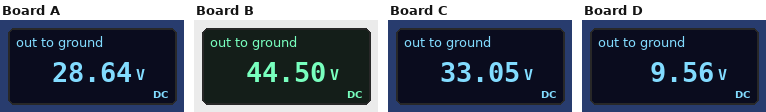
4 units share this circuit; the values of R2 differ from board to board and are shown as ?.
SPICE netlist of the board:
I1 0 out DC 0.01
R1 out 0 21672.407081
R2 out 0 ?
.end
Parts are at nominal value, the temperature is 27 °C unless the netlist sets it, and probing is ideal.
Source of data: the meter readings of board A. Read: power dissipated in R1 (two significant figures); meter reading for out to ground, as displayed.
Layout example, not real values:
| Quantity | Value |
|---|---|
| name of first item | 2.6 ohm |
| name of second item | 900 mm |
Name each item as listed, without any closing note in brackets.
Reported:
| Quantity | Value |
|---|---|
| power dissipated in R1 | 38 mW |
| meter reading for out to ground, as displayed | 28.64 V |
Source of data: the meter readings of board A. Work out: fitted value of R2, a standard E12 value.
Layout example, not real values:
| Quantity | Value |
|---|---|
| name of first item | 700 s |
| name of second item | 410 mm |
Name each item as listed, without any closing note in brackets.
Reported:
| Quantity | Value |
|---|---|
| fitted value of R2, a standard E12 value | 3.3 kΩ |
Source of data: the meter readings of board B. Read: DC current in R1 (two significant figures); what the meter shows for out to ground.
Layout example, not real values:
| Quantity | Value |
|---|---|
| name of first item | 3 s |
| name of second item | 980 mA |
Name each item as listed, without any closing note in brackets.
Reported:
| Quantity | Value |
|---|---|
| DC current in R1 | 2.1 mA |
| what the meter shows for out to ground | 44.50 V |
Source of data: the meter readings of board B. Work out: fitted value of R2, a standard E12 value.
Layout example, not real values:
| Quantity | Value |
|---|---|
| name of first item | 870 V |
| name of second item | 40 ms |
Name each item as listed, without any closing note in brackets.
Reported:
| Quantity | Value |
|---|---|
| fitted value of R2, a standard E12 value | 5.6 kΩ |
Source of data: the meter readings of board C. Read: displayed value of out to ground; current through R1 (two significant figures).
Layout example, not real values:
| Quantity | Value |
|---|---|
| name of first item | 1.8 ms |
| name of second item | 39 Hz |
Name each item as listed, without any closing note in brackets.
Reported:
| Quantity | Value |
|---|---|
| displayed value of out to ground | 33.05 V |
| current through R1 | 1.5 mA |
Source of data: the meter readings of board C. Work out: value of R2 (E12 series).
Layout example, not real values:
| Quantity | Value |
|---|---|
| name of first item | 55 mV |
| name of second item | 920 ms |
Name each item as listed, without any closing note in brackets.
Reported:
| Quantity | Value |
|---|---|
| value of R2 | 3.9 kΩ |
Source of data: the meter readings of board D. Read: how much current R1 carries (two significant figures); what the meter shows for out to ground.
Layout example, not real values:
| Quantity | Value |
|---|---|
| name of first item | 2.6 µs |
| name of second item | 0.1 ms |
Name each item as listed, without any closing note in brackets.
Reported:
| Quantity | Value |
|---|---|
| how much current R1 carries | 440 µA |
| what the meter shows for out to ground | 9.56 V |
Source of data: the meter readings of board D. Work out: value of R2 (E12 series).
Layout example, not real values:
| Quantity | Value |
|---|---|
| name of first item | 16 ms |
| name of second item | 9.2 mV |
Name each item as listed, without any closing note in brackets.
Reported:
| Quantity | Value |
|---|---|
| value of R2 | 1 kΩ |
